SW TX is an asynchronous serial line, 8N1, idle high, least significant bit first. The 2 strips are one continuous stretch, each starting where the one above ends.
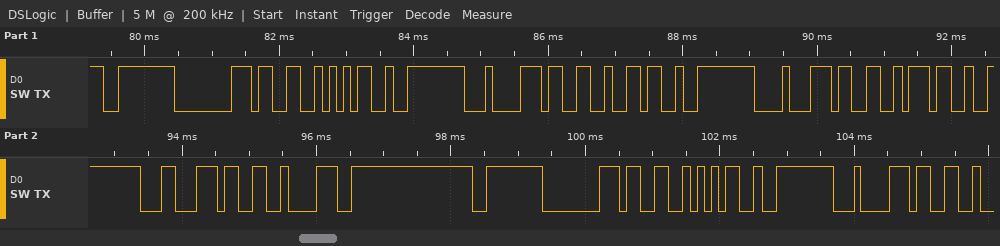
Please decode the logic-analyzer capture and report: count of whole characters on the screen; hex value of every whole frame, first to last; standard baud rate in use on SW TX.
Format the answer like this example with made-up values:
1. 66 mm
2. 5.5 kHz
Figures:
1. 23
2. FE 80 33 35 FE 84 33 36 FE 88 33 37 FE 8C 33 38 FE 80 33 35 FE 84 33
3. 9600 baud
